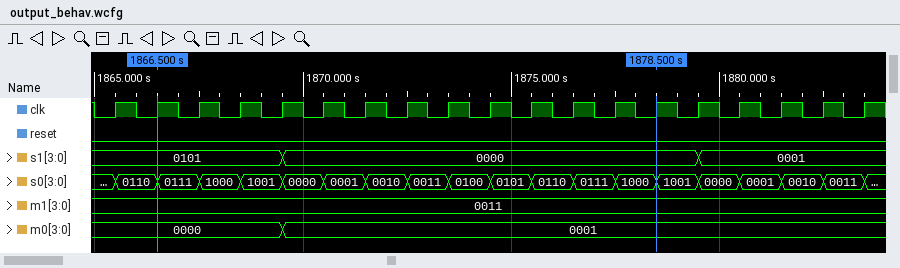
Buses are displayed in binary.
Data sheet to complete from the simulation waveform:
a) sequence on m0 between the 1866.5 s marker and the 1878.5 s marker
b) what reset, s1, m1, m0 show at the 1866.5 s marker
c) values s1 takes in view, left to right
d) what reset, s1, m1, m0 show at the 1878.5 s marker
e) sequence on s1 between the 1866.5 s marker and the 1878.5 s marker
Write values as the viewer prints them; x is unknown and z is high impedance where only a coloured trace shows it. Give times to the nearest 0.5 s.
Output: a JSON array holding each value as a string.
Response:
["0000, 0001", "reset=0, s1=0101, m1=0011, m0=0000", "0101, 0000, 0001", "reset=0, s1=0000, m1=0011, m0=0001", "0101, 0000"]
